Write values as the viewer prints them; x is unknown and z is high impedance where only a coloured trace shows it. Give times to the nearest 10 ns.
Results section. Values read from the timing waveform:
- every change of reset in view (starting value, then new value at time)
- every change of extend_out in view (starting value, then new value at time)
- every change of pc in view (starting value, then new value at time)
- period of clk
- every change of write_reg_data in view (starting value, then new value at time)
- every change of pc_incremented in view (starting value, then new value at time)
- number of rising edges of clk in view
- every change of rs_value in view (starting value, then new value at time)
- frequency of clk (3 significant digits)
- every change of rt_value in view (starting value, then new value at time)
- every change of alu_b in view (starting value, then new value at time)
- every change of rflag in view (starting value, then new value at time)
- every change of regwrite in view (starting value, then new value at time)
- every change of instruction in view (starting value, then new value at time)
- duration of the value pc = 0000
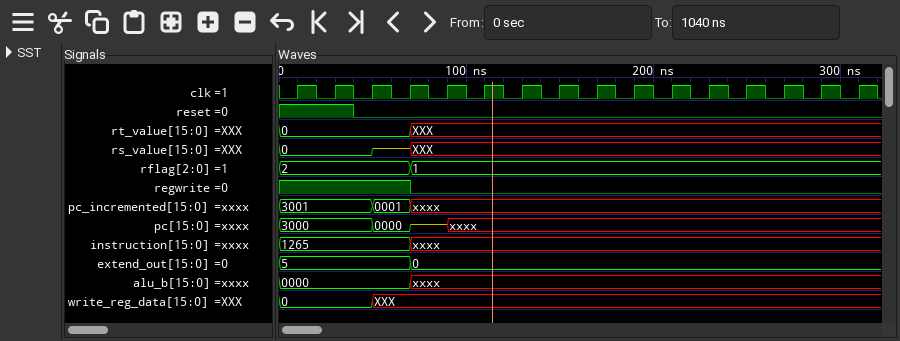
1, 0 at 40 ns
5, 0 at 70 ns
3000, 0000 at 50 ns, z at 70 ns, xxxx at 90 ns
20 ns
0, XXX at 50 ns
3001, 0001 at 50 ns, xxxx at 70 ns
16
0, z at 50 ns, XXX at 70 ns
50.0 MHz
0, XXX at 70 ns
0000, xxxx at 70 ns
2, 1 at 70 ns
1, 0 at 70 ns
1265, xxxx at 70 ns
20 ns
